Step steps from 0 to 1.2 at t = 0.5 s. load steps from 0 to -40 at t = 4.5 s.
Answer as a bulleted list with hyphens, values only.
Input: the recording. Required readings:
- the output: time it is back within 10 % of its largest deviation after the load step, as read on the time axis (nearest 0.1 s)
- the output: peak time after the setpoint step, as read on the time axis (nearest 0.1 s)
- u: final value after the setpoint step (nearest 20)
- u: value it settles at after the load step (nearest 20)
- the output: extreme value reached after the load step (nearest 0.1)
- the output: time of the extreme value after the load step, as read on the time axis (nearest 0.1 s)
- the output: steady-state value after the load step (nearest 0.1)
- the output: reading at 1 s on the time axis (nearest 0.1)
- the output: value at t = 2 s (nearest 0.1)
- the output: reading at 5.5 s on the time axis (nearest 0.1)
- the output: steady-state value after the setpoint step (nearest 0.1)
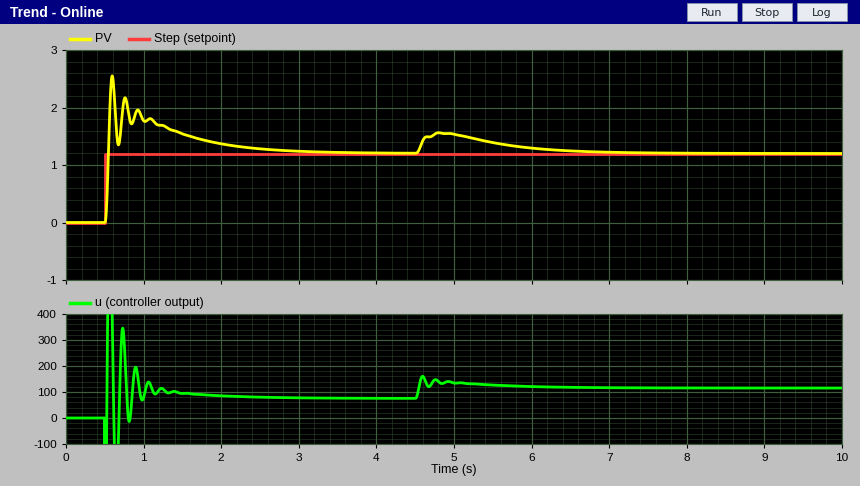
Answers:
- 6.7 s
- 0.6 s
- 80
- 120
- 1.6
- 4.8 s
- 1.2
- 1.8
- 1.4
- 1.4
- 1.2
